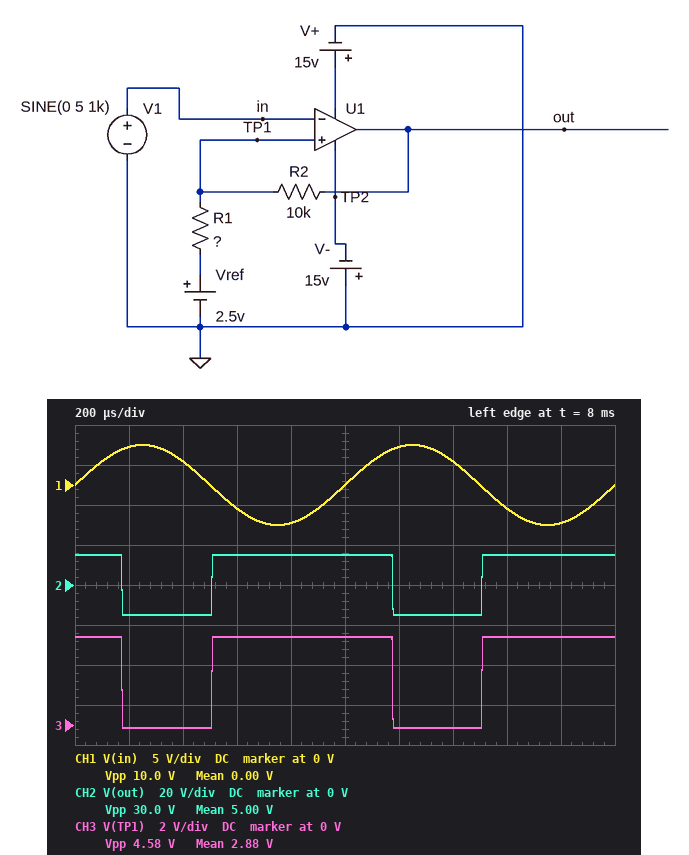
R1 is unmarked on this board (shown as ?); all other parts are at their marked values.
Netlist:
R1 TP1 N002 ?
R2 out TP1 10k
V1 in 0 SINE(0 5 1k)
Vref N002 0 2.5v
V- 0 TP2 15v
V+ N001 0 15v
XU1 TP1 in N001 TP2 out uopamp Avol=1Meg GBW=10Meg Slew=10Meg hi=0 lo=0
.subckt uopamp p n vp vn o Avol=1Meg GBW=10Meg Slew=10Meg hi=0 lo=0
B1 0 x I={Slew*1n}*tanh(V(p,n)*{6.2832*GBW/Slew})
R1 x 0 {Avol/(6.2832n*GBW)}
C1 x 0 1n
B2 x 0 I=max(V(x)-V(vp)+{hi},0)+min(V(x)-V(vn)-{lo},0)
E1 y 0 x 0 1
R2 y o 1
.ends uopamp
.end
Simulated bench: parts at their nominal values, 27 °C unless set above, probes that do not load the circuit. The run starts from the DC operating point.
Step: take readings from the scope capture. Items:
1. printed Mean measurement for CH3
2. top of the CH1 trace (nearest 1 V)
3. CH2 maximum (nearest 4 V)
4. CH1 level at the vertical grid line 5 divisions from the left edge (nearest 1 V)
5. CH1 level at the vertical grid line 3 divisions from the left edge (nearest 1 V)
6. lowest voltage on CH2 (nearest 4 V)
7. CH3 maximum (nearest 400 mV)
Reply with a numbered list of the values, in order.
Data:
1. 2.88 V
2. 5 V
3. 16 V
4. 0 V
5. -3 V
6. -16 V
7. 4.4 V
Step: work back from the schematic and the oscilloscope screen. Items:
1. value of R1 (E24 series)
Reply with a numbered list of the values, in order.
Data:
1. 1.8 kΩ
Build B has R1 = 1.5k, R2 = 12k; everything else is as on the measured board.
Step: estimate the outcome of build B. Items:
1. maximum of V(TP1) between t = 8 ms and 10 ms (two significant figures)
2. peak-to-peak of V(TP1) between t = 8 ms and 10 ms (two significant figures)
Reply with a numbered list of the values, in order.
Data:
1. 3.9 V
2. 3.3 V
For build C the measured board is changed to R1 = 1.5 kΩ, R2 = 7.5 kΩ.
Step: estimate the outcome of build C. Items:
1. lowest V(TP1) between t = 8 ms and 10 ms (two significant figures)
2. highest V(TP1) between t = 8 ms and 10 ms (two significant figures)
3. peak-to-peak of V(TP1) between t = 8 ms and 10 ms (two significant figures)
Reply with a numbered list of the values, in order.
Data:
1. -420 mV
2. 4.6 V
3. 5.0 V
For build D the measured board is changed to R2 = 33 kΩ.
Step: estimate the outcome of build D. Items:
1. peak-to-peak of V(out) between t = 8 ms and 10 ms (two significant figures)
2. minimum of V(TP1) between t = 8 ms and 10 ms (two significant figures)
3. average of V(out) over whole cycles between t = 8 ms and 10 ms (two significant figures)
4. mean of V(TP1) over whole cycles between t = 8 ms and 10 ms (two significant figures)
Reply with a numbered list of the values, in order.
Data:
1. 30 V
2. 1.6 V
3. 4.8 V
4. 2.6 V
